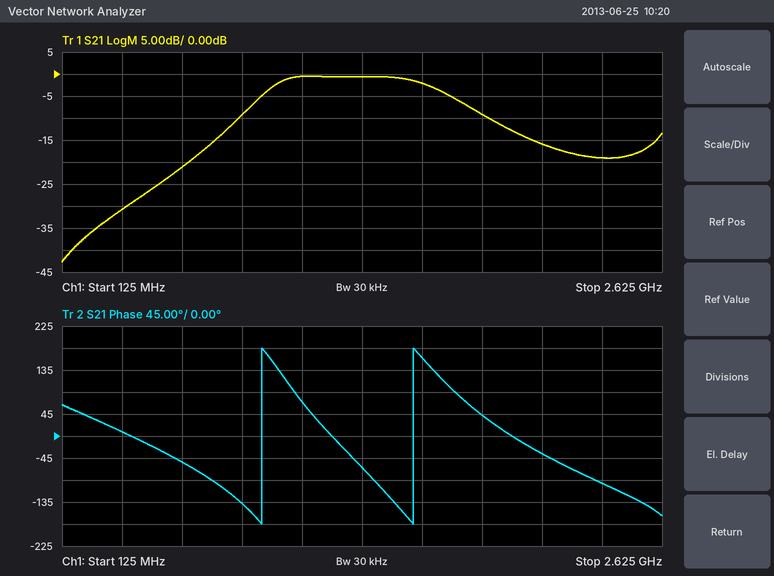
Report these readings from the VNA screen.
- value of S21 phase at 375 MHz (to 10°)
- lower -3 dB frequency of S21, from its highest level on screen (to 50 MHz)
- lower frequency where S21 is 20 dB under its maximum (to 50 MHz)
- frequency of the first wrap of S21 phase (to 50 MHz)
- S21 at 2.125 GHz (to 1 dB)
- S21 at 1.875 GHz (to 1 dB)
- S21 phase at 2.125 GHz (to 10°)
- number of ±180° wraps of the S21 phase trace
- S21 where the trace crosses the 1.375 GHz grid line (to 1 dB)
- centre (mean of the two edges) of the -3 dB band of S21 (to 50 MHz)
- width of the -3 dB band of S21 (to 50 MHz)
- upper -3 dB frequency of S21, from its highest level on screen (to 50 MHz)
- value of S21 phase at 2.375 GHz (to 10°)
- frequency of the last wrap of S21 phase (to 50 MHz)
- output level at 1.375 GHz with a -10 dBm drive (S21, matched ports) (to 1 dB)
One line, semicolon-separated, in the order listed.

10°; 1.00 GHz; 650 MHz; 950 MHz; -16 dB; -9 dB; -40°; 2; -1 dB; 1.35 GHz; 700 MHz; 1.70 GHz; -100°; 1.60 GHz; -11 dBm
